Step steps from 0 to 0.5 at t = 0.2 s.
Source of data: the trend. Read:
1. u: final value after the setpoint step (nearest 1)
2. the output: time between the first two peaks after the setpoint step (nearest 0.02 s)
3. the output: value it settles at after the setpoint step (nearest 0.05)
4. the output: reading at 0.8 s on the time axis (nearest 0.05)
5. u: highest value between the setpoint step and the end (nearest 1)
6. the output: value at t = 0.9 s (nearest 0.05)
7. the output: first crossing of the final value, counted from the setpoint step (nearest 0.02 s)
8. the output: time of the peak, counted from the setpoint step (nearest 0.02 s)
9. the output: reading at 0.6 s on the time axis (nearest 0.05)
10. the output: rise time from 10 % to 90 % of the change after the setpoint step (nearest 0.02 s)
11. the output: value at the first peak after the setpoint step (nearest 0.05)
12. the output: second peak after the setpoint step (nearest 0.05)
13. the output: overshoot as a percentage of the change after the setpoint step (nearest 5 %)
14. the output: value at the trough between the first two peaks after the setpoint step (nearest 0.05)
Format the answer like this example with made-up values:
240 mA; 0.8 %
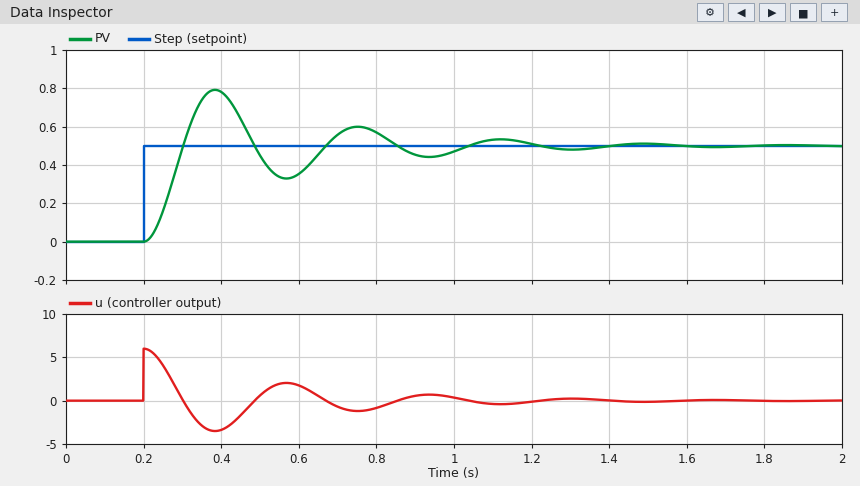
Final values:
0; 0.36 s; 0.50; 0.55; 6; 0.45; 0.10 s; 0.18 s; 0.35; 0.06 s; 0.80; 0.60; 60 %; 0.35
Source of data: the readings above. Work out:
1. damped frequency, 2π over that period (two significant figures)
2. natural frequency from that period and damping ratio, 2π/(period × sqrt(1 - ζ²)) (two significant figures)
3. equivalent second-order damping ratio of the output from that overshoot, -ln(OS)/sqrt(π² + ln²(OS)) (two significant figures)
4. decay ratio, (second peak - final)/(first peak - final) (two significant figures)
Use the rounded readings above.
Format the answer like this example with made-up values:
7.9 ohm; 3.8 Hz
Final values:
17 rad/s; 18 rad/s; 0.16; 0.33
